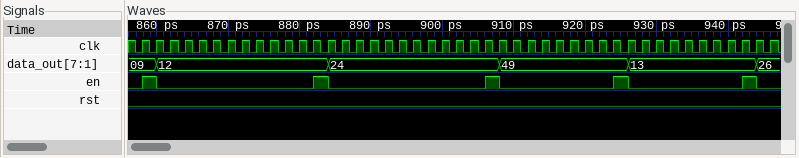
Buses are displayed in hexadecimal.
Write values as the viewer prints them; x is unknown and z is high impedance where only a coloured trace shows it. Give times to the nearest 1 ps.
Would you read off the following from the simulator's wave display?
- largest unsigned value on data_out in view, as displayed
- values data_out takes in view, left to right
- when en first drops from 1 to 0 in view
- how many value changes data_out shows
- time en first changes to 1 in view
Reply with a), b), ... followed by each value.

a) 49
b) 09, 12, 24, 49, 13, 26
c) 860 ps
d) 5
e) 858 ps
